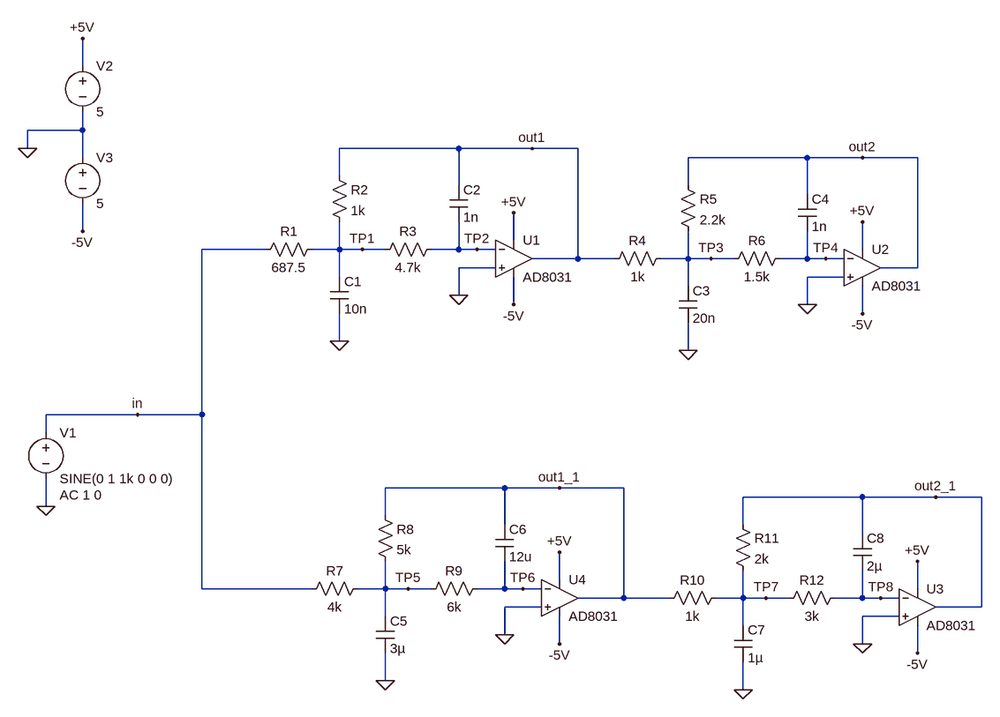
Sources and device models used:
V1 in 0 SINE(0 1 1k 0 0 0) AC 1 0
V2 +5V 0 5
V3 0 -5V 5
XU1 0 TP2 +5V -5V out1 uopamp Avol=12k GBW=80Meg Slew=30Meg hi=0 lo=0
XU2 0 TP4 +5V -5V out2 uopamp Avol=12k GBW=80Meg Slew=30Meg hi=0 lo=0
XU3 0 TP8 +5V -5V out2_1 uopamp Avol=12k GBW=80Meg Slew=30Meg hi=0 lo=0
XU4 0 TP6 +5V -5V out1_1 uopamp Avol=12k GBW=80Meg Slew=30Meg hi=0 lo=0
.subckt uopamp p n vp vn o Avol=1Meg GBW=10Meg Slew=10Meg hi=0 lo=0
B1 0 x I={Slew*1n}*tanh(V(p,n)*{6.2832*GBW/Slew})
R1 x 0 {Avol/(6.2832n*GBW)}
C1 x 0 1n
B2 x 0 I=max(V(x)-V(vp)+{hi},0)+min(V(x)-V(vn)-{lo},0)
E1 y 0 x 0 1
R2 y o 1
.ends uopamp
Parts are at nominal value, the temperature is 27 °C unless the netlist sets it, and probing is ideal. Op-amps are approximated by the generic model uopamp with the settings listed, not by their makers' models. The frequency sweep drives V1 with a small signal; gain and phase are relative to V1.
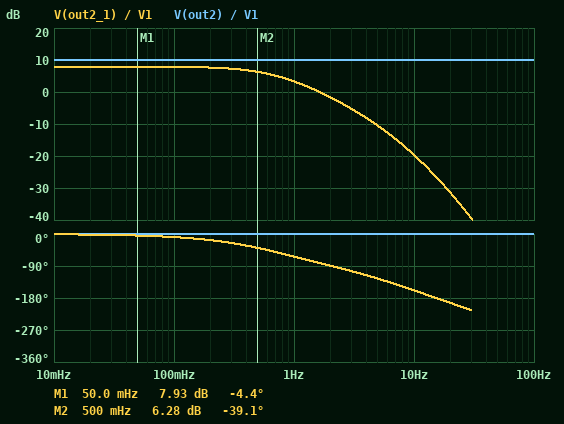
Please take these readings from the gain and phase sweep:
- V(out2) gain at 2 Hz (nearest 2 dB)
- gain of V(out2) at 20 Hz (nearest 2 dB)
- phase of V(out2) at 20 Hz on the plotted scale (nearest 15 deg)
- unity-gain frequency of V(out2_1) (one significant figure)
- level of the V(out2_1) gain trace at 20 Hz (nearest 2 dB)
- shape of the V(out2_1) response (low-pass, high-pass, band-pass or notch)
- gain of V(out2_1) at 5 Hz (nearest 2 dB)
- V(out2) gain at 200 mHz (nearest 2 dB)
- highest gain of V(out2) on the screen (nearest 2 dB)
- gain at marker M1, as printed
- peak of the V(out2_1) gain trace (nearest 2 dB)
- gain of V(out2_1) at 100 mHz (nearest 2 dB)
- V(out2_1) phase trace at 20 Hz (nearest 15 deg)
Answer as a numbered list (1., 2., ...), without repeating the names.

1. 10 dB
2. 10 dB
3. 0 deg
4. 2 Hz
5. -32 dB
6. low-pass
7. -10 dB
8. 10 dB
9. 10 dB
10. 7.93 dB
11. 8 dB
12. 8 dB
13. -195 deg
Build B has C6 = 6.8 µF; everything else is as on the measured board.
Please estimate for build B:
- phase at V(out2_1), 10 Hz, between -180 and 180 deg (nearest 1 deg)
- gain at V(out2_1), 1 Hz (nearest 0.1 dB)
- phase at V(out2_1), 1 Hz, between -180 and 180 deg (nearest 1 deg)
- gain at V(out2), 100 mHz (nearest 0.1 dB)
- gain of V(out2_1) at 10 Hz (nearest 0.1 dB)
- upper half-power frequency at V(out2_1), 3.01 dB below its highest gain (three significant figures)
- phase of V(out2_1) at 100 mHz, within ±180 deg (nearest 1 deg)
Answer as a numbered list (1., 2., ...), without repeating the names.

1. -156 deg
2. 5.9 dB
3. -47 deg
4. 10.1 dB
5. -14.6 dB
6. 1.28 Hz
7. -5 deg
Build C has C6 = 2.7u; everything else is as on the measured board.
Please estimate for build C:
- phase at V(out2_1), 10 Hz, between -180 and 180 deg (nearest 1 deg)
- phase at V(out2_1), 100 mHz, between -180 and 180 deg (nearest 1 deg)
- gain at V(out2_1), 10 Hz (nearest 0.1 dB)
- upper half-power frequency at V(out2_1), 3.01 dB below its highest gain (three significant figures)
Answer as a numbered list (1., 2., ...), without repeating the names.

1. -145 deg
2. -3 deg
3. -6.5 dB
4. 3.00 Hz
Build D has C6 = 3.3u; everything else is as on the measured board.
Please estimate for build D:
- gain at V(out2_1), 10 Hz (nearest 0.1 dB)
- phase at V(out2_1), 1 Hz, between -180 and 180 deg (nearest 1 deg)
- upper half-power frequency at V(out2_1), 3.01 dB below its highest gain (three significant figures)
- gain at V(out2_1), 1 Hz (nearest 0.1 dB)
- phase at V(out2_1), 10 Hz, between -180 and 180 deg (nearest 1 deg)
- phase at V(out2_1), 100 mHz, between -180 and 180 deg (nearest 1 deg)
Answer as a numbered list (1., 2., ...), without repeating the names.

1. -8.2 dB
2. -29 deg
3. 2.52 Hz
4. 7.4 dB
5. -148 deg
6. -3 deg
